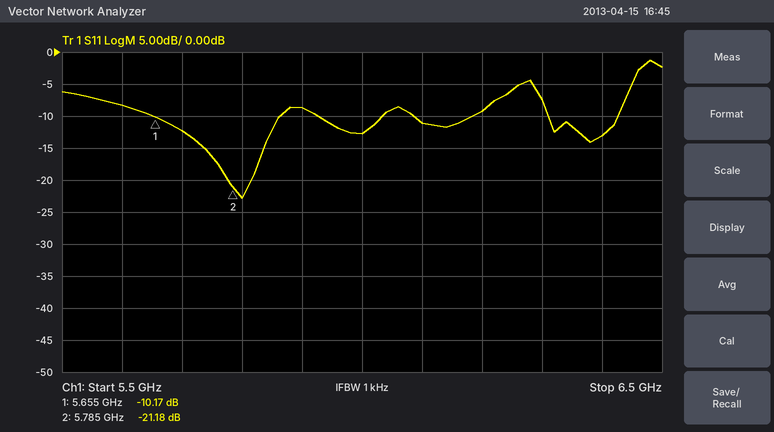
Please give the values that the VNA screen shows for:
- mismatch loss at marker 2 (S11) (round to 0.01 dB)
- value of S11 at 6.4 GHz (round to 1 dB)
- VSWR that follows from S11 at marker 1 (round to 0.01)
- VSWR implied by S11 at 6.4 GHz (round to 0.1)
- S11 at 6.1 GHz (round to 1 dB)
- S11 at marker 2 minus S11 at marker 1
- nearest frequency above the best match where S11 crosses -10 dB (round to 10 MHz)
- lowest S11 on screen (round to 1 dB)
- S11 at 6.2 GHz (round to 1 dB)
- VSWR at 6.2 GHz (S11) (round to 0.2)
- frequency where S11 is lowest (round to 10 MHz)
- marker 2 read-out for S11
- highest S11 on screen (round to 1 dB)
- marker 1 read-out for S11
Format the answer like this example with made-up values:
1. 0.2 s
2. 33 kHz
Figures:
1. 0.03 dB
2. -13 dB
3. 1.90
4. 1.6
5. -11 dB
6. -11.01 dB
7. 5.86 GHz
8. -23 dB
9. -9 dB
10. 2.0
11. 5.80 GHz
12. -21.18 dB
13. -1 dB
14. -10.17 dB
